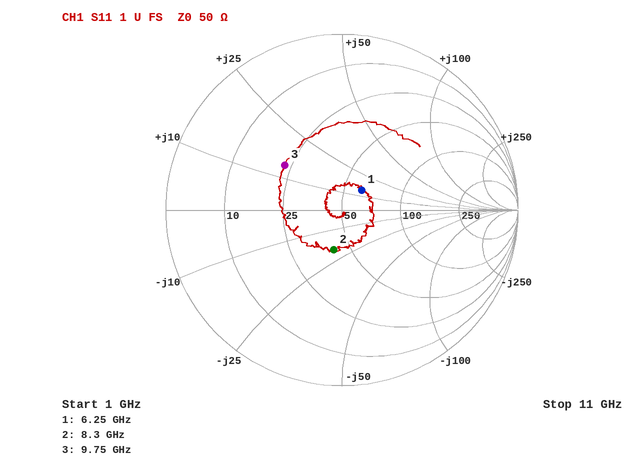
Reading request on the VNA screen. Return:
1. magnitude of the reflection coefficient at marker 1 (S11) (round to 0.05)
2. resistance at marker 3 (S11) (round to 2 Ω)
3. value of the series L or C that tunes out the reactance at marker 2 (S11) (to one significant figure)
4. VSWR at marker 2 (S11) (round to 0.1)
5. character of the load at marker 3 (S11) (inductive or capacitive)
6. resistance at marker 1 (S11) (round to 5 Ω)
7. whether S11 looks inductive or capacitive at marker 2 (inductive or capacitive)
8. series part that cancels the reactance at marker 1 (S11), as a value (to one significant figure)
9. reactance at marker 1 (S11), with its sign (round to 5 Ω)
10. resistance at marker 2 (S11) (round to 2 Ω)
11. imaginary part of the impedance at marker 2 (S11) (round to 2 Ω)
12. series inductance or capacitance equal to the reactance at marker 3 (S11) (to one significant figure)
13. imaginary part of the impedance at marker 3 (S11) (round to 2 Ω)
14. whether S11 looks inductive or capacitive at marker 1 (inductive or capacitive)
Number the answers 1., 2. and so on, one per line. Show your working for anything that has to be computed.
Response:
1. 0.15
2. 22 Ω
3. L = 20 Ω/(2π × 8.3 GHz) ≈ 384 pH, so 400 pH to one significant figure
4. 1.6
5. inductive
6. 60 Ω
7. capacitive
8. C = 1/(2π × 6.25 GHz × 15 Ω) ≈ 2 pF
9. +15 Ω
10. 42 Ω
11. -20 Ω
12. L = 14 Ω/(2π × 9.75 GHz) ≈ 229 pH, so 200 pH to one significant figure
13. +14 Ω
14. inductive
